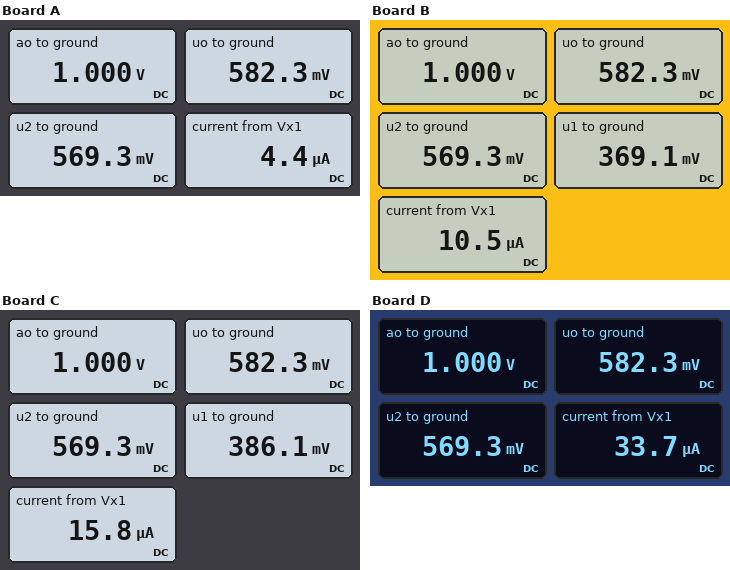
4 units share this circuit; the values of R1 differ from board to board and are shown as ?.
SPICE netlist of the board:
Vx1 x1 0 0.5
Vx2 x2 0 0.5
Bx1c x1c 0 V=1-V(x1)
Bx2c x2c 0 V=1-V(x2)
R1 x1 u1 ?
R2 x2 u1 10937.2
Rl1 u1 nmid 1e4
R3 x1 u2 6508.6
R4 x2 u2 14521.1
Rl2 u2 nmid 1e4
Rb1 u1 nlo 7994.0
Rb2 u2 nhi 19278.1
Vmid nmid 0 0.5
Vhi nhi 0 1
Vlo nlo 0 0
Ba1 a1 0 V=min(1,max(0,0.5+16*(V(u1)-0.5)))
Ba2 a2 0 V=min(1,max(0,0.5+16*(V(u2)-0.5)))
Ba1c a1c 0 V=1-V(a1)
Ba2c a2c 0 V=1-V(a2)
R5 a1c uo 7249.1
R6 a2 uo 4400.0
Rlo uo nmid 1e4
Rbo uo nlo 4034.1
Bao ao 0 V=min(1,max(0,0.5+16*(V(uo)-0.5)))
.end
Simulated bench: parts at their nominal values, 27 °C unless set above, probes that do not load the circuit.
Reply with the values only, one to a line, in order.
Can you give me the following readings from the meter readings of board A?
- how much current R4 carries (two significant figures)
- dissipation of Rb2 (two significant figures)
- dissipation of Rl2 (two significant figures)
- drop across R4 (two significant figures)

4.8 µA
9.6 µW
480 nW
69 mV
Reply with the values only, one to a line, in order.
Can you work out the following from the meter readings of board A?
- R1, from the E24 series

10 kΩ
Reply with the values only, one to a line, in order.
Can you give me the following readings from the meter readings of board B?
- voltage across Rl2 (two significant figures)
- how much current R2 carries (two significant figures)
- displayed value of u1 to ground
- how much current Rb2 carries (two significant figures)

69 mV
12 µA
369.1 mV
22 µA
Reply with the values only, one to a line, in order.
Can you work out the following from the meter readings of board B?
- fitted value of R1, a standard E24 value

6.2 kΩ
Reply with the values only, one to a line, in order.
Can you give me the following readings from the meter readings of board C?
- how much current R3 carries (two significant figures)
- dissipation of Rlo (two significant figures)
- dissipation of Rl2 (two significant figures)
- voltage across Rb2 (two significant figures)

11 µA
680 nW
480 nW
430 mV
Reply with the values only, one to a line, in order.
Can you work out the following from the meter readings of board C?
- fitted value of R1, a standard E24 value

4.3 kΩ
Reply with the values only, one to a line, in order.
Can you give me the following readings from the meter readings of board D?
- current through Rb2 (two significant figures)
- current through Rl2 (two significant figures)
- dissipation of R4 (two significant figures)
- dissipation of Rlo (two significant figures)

22 µA
6.9 µA
330 nW
680 nW
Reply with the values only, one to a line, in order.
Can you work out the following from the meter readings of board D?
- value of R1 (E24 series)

1.3 kΩ
